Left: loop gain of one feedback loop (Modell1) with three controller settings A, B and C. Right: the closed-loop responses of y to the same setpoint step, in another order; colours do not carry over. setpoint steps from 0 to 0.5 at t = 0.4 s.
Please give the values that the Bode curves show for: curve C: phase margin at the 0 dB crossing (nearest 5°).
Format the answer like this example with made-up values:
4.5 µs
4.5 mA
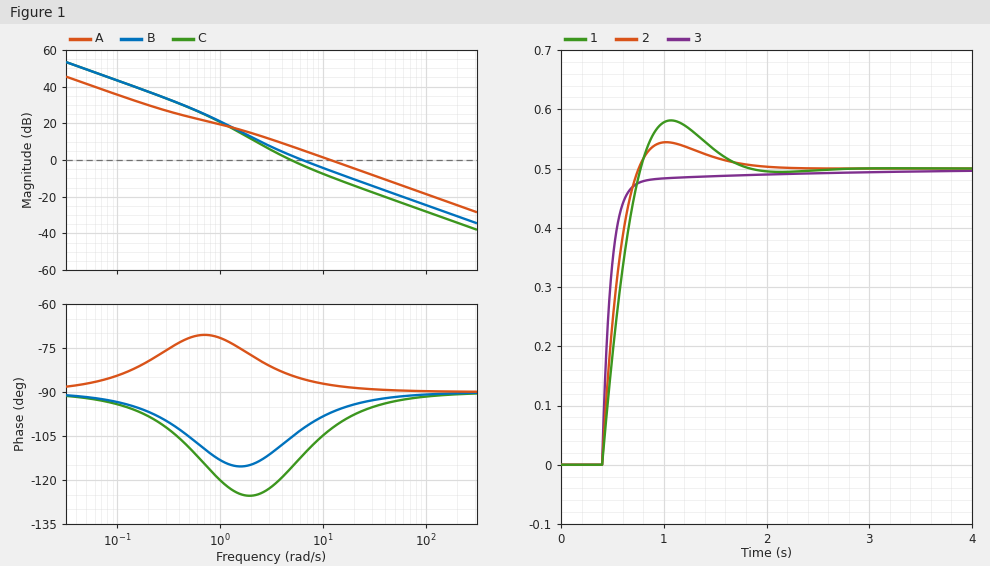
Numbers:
65°
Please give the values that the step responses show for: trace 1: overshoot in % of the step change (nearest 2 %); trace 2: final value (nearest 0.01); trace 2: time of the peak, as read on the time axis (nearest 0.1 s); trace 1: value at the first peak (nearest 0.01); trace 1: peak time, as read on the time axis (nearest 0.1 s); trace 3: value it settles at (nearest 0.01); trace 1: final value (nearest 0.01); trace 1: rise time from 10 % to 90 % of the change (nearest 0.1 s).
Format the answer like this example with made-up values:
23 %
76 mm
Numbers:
16 %
0.50
1.0 s
0.58
1.1 s
0.50
0.50
0.3 s
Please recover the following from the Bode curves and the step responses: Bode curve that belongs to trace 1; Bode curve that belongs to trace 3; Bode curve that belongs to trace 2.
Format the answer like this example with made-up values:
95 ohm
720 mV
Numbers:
C
A
B
